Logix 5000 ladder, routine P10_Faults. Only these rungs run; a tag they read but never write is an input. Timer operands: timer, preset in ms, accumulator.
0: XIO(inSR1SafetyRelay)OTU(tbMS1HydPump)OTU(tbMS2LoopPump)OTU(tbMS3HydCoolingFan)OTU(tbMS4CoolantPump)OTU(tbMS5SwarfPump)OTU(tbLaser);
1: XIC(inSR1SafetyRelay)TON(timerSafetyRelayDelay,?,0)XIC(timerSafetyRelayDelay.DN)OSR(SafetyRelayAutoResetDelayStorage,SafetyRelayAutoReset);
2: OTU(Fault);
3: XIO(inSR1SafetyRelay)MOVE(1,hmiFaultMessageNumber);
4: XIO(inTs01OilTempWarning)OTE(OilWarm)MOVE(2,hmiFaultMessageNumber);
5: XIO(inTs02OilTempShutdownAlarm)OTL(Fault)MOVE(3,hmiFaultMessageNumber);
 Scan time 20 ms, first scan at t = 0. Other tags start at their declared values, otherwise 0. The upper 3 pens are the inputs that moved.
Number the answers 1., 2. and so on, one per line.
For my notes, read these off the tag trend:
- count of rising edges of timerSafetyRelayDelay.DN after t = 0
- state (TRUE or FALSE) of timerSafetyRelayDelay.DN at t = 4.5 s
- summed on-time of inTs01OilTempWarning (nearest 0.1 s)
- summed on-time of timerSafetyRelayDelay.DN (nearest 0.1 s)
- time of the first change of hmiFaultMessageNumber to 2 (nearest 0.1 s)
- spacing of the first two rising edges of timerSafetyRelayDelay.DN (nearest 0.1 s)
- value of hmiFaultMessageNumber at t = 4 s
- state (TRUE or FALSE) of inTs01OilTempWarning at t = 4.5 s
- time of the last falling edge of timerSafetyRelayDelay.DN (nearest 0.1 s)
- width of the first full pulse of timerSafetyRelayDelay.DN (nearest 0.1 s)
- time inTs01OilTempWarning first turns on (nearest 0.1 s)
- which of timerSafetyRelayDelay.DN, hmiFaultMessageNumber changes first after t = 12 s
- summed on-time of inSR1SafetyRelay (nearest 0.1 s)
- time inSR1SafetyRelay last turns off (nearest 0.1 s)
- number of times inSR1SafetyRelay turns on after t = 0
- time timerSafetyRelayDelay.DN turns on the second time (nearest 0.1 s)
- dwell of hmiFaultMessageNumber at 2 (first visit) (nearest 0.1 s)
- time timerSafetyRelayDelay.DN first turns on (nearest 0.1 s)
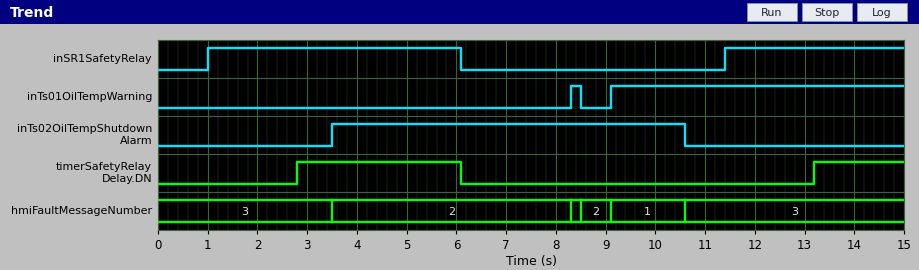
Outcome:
1. 2
2. TRUE
3. 6.1 s
4. 5.1 s
5. 3.5 s
6. 10.4 s
7. 2
8. FALSE
9. 6.1 s
10. 3.3 s
11. 8.3 s
12. timerSafetyRelayDelay.DN
13. 8.7 s
14. 6.1 s
15. 2
16. 13.2 s
17. 4.8 s
18. 2.8 s
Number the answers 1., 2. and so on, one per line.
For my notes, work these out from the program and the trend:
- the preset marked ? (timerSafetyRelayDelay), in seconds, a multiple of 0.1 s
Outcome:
1. 1.8 s
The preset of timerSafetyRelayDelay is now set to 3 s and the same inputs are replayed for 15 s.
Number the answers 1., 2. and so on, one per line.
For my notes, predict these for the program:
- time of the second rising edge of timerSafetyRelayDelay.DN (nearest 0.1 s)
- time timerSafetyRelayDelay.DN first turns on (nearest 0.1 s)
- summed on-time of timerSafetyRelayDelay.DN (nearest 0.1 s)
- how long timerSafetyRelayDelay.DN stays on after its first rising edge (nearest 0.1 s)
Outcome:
1. 14.4 s
2. 4.0 s
3. 2.7 s
4. 2.1 s
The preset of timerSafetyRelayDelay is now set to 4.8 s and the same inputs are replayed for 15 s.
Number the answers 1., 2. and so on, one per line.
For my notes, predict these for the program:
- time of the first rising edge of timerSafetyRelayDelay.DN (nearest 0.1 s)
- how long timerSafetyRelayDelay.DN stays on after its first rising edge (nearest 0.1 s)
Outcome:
1. 5.8 s
2. 0.3 s
